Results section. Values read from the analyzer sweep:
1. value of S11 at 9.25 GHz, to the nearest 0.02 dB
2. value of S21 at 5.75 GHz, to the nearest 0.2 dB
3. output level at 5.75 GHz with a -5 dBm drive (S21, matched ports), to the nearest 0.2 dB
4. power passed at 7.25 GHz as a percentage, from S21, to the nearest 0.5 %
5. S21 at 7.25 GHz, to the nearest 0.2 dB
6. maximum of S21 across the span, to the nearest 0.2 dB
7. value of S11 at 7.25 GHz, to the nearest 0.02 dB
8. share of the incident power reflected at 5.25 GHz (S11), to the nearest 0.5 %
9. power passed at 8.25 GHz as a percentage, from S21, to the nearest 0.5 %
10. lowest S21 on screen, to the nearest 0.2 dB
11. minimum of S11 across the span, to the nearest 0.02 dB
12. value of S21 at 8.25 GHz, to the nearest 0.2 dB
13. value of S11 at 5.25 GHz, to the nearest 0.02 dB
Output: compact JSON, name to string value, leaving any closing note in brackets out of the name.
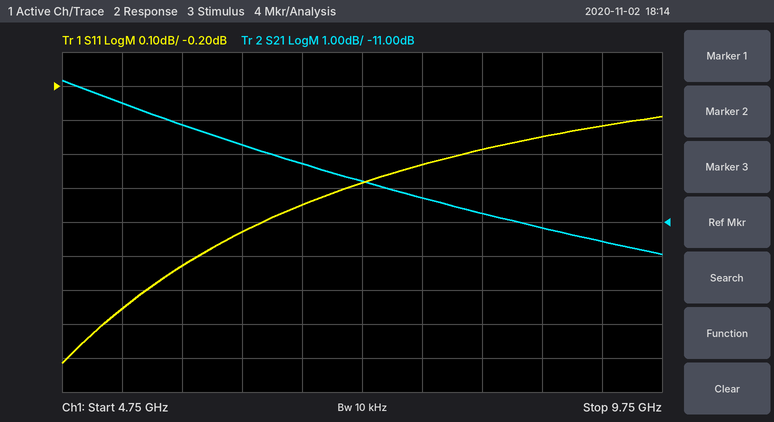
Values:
{"value of S11 at 9.25 GHz, to the nearest 0.02 dB": "-0.32 dB", "value of S21 at 5.75 GHz, to the nearest 0.2 dB": "-8.2 dB", "output level at 5.75 GHz with a -5 dBm drive (S21, matched ports), to the nearest 0.2 dB": "-13.2 dBm", "power passed at 7.25 GHz as a percentage, from S21, to the nearest 0.5 %": "10.5 %", "S21 at 7.25 GHz, to the nearest 0.2 dB": "-9.8 dB", "maximum of S21 across the span, to the nearest 0.2 dB": "-6.8 dB", "value of S11 at 7.25 GHz, to the nearest 0.02 dB": "-0.48 dB", "share of the incident power reflected at 5.25 GHz (S11), to the nearest 0.5 %": "82.0 %", "power passed at 8.25 GHz as a percentage, from S21, to the nearest 0.5 %": "8.5 %", "lowest S21 on screen, to the nearest 0.2 dB": "-12.0 dB", "minimum of S11 across the span, to the nearest 0.02 dB": "-1.02 dB", "value of S21 at 8.25 GHz, to the nearest 0.2 dB": "-10.8 dB", "value of S11 at 5.25 GHz, to the nearest 0.02 dB": "-0.86 dB"}
